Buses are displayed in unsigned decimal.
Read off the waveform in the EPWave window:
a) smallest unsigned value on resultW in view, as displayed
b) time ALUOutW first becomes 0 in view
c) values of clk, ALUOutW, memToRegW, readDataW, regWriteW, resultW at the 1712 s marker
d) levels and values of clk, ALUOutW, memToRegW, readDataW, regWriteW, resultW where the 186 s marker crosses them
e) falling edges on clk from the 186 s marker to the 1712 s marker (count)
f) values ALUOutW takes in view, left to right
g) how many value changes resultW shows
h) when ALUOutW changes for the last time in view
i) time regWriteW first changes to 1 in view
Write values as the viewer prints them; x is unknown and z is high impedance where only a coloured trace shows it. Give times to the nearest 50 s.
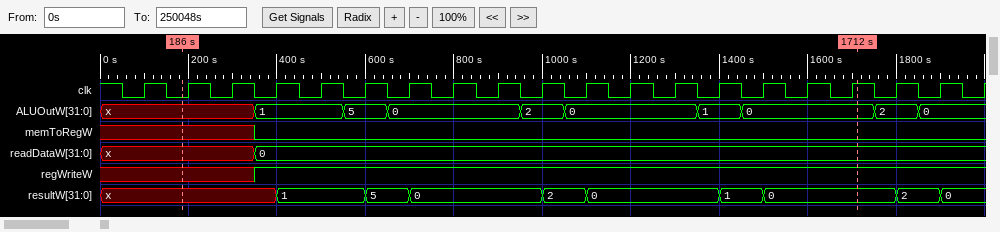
0
650 s
clk=1, ALUOutW=0, memToRegW=0, readDataW=0, regWriteW=1, resultW=0
clk=0, ALUOutW=x, memToRegW=x, readDataW=x, regWriteW=x, resultW=x
15
x, 1, 5, 0, 2, 0, 1, 0, 2, 0
9
1850 s
350 s
